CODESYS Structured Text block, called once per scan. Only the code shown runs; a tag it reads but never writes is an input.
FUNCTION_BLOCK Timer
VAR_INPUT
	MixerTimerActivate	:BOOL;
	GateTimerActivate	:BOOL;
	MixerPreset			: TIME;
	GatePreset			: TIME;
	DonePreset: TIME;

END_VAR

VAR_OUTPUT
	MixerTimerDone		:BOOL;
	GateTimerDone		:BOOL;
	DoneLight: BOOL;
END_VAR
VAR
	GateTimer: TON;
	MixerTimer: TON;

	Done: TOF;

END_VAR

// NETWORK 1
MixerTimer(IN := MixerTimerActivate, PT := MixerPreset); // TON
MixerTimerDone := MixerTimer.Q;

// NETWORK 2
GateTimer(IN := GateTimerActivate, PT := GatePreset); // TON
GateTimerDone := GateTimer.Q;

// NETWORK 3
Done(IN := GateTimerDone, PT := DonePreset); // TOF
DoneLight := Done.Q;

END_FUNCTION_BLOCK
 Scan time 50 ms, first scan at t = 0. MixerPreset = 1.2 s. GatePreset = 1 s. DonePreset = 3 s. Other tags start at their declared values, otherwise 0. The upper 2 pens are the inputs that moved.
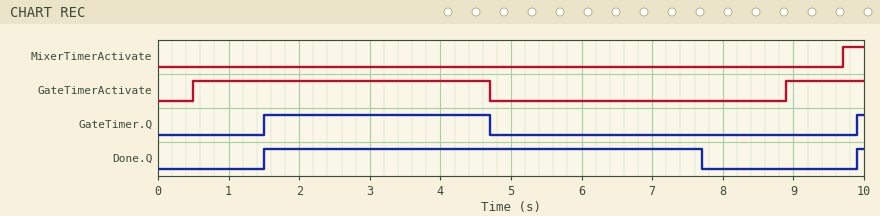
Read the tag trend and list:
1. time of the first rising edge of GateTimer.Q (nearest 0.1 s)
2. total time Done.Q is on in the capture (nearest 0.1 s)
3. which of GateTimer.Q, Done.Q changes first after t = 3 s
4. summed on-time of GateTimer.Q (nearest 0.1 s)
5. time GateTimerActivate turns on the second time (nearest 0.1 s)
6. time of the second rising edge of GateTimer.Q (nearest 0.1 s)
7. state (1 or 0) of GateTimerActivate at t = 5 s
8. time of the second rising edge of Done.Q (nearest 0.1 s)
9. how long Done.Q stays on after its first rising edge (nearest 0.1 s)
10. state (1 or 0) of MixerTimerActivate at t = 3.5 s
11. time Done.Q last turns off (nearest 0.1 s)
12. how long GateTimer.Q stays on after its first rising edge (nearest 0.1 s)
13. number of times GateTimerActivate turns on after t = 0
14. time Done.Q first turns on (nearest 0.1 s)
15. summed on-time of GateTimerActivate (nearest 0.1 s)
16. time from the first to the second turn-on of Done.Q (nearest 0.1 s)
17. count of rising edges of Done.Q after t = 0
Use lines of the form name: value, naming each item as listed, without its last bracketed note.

time of the first rising edge of GateTimer.Q: 1.5 s
total time Done.Q is on in the capture: 6.3 s
which of GateTimer.Q, Done.Q changes first after t = 3 s: GateTimer.Q
summed on-time of GateTimer.Q: 3.3 s
time GateTimerActivate turns on the second time: 8.9 s
time of the second rising edge of GateTimer.Q: 9.9 s
state (1 or 0) of GateTimerActivate at t = 5 s: 0
time of the second rising edge of Done.Q: 9.9 s
how long Done.Q stays on after its first rising edge: 6.2 s
state (1 or 0) of MixerTimerActivate at t = 3.5 s: 0
time Done.Q last turns off: 7.7 s
how long GateTimer.Q stays on after its first rising edge: 3.2 s
number of times GateTimerActivate turns on after t = 0: 2
time Done.Q first turns on: 1.5 s
summed on-time of GateTimerActivate: 5.3 s
time from the first to the second turn-on of Done.Q: 8.4 s
count of rising edges of Done.Q after t = 0: 2
